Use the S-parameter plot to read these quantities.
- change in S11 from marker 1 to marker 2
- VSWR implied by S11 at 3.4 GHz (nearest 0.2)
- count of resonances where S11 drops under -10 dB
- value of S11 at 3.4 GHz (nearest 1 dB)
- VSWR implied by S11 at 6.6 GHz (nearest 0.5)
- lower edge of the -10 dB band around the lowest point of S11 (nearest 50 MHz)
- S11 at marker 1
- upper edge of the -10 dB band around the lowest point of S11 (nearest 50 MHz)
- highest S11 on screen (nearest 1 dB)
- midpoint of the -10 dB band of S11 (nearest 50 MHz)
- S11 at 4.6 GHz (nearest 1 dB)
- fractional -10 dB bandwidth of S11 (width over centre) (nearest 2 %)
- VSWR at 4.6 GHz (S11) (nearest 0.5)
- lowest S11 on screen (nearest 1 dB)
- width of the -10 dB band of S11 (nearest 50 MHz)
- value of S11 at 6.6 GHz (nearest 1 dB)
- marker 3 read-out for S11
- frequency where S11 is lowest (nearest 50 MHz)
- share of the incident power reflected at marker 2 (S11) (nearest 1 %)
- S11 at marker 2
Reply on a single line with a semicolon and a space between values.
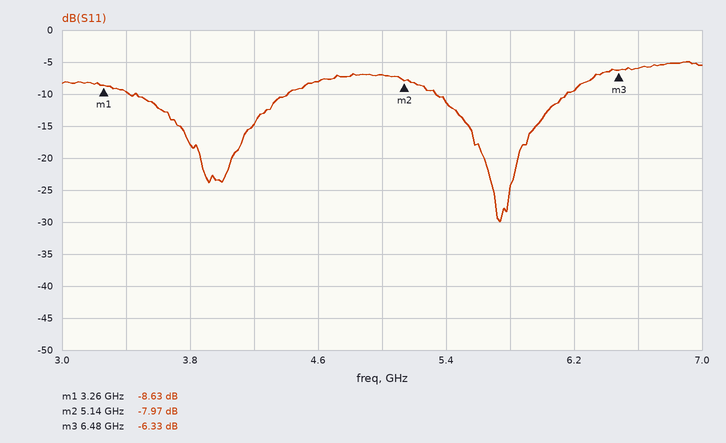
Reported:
0.66 dB; 2.0; 2; -10 dB; 3.0; 5.35 GHz; -8.63 dB; 6.15 GHz; -5 dB; 5.75 GHz; -8 dB; 14 %; 2.5; -30 dB; 800 MHz; -6 dB; -6.33 dB; 5.75 GHz; 16 %; -7.97 dB
